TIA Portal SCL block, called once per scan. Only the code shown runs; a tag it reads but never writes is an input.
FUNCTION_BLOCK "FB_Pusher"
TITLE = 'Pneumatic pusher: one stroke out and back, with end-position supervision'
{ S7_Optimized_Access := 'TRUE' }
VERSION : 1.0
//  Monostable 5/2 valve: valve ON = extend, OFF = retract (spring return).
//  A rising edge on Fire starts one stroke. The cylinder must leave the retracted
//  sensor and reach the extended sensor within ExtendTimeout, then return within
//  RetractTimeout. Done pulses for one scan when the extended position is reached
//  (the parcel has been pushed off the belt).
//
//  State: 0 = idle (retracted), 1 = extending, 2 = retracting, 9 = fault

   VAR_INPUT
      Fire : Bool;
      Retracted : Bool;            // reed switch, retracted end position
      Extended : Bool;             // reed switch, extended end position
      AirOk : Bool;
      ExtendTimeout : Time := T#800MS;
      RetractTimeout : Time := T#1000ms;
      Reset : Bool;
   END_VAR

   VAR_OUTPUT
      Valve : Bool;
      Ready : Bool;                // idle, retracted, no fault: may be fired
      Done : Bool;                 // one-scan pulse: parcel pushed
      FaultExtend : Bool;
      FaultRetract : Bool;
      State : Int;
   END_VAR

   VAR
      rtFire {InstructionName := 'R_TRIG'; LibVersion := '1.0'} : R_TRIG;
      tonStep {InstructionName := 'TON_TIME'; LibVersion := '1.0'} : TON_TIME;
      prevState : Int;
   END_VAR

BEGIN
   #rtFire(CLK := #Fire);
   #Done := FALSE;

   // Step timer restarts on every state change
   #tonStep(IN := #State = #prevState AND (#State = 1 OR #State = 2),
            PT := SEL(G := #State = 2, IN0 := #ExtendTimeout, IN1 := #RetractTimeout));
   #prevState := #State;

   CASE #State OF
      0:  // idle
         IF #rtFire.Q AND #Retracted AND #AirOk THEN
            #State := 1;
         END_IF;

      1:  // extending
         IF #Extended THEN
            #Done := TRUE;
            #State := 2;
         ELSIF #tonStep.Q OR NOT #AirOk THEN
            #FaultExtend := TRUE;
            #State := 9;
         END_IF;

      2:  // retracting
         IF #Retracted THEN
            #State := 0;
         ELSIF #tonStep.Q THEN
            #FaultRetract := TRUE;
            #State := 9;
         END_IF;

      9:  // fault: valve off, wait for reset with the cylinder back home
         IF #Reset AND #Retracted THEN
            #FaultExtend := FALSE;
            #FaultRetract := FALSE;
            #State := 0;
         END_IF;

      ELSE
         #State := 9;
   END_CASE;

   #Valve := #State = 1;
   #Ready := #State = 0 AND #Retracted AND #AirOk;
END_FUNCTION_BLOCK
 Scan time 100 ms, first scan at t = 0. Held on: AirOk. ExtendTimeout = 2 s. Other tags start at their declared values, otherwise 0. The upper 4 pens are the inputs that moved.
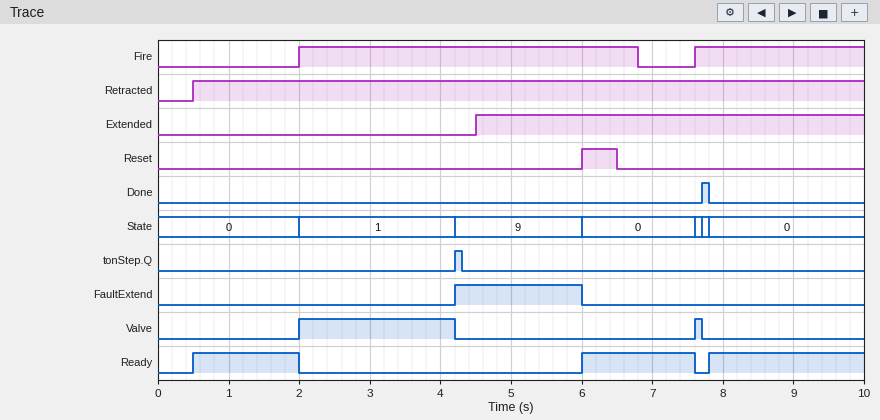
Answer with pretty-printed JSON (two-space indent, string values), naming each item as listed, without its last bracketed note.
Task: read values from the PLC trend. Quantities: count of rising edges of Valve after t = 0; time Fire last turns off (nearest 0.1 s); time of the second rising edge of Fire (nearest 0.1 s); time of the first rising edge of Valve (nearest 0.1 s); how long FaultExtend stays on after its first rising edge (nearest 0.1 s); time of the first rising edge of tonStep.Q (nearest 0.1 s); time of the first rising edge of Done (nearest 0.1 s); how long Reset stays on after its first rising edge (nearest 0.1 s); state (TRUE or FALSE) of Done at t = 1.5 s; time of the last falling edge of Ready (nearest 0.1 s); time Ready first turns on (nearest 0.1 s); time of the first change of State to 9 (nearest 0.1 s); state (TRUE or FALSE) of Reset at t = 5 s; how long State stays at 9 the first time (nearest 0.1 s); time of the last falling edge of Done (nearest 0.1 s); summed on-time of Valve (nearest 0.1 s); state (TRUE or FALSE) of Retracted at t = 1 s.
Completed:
{
  "count of rising edges of Valve after t = 0": "2",
  "time Fire last turns off": "6.8 s",
  "time of the second rising edge of Fire": "7.6 s",
  "time of the first rising edge of Valve": "2.0 s",
  "how long FaultExtend stays on after its first rising edge": "1.8 s",
  "time of the first rising edge of tonStep.Q": "4.2 s",
  "time of the first rising edge of Done": "7.7 s",
  "how long Reset stays on after its first rising edge": "0.5 s",
  "state (TRUE or FALSE) of Done at t = 1.5 s": "FALSE",
  "time of the last falling edge of Ready": "7.6 s",
  "time Ready first turns on": "0.5 s",
  "time of the first change of State to 9": "4.2 s",
  "state (TRUE or FALSE) of Reset at t = 5 s": "FALSE",
  "how long State stays at 9 the first time": "1.8 s",
  "time of the last falling edge of Done": "7.8 s",
  "summed on-time of Valve": "2.3 s",
  "state (TRUE or FALSE) of Retracted at t = 1 s": "TRUE"
}
